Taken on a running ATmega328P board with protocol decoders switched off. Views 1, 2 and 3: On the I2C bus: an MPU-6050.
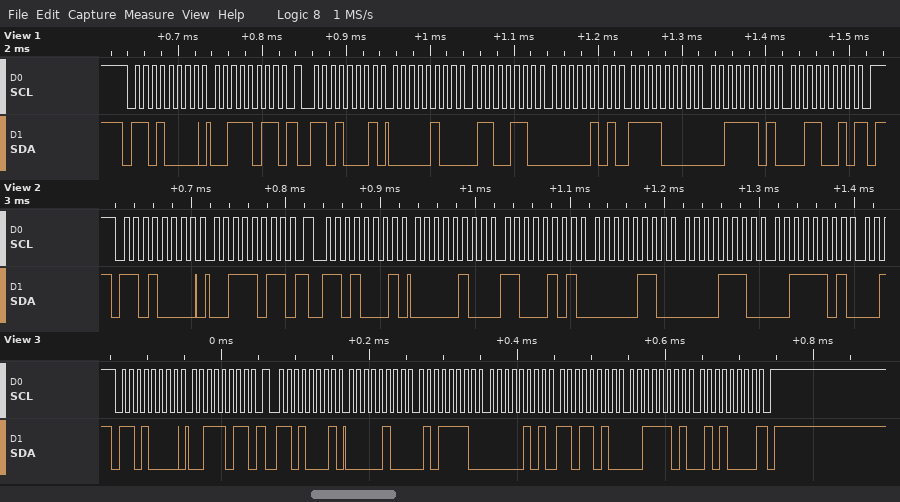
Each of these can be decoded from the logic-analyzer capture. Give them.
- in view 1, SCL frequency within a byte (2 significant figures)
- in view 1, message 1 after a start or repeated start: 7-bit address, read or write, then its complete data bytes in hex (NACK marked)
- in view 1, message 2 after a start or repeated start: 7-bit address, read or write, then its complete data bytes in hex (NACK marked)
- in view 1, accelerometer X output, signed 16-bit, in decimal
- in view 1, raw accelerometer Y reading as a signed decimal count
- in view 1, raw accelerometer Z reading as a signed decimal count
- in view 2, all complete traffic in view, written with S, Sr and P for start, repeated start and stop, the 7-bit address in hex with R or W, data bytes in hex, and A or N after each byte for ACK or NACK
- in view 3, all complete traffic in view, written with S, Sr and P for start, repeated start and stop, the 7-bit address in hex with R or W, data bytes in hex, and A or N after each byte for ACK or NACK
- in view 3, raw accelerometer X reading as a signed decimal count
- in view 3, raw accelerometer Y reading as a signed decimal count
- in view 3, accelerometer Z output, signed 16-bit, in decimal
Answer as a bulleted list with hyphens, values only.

- 100 kHz
- 0x68 write: 3B
- 0x68 read: 04 66 05 F0 3D 32 NACK
- 1126
- 1520
- 15666
- S 68W A 3B A Sr 68R A 04 A C5 A 06 A 0E A 3D A
- S 68W A 3B A Sr 68R A 04 A 5E A 05 A DA A 3D A 50 N P
- 1118
- 1498
- 15696
